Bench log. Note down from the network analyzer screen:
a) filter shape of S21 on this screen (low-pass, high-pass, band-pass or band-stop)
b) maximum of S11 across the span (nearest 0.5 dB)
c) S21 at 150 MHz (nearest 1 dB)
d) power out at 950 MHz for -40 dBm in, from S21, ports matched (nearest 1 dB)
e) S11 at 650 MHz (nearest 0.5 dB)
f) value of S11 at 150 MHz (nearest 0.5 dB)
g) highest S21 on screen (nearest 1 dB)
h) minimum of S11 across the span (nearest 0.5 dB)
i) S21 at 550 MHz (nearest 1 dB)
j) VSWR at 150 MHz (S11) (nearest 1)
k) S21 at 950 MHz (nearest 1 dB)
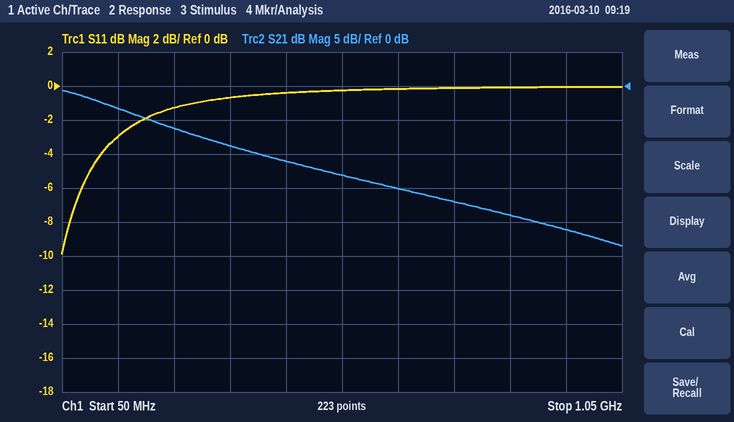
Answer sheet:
low-pass
0.0 dB
-3 dB
-61 dBm
0.0 dB
-3.0 dB
-1 dB
-10.0 dB
-13 dB
6
-21 dB
